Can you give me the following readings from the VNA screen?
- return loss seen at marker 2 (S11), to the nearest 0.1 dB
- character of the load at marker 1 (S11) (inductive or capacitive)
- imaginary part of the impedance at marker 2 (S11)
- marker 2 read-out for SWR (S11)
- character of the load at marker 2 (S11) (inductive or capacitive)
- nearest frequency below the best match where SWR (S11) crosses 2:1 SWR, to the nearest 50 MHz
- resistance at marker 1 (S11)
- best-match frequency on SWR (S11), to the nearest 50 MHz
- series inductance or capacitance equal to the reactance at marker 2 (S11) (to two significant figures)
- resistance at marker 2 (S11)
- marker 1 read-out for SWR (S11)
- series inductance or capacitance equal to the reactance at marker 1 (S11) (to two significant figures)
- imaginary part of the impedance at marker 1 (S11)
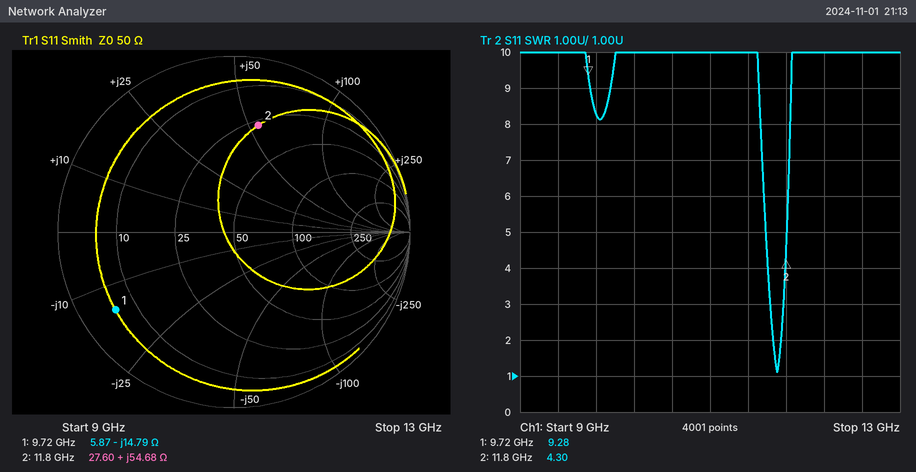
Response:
4.1 dB
capacitive
+54.68 Ω
4.30
inductive
11.65 GHz
5.87 Ω
11.70 GHz
740 pH
27.60 Ω
9.28
1.1 pF
-14.79 Ω
